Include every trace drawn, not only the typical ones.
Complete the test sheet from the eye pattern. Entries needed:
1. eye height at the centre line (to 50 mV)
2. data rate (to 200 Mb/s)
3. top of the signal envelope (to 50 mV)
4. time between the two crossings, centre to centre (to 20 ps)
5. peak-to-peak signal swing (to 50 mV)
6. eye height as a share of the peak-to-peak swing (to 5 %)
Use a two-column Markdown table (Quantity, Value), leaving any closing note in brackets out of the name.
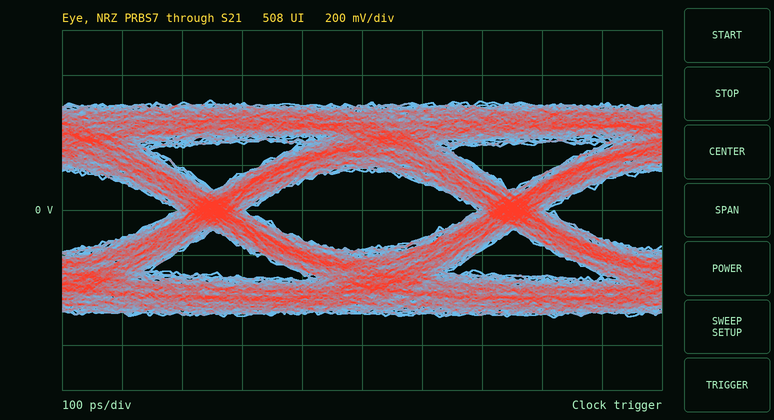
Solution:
| Quantity | Value |
|---|---|
| eye height at the centre line | 350 mV |
| data rate | 2.0 Gb/s |
| top of the signal envelope | 500 mV |
| time between the two crossings, centre to centre | 500 ps |
| peak-to-peak signal swing | 950 mV |
| eye height as a share of the peak-to-peak swing | 35 % |
